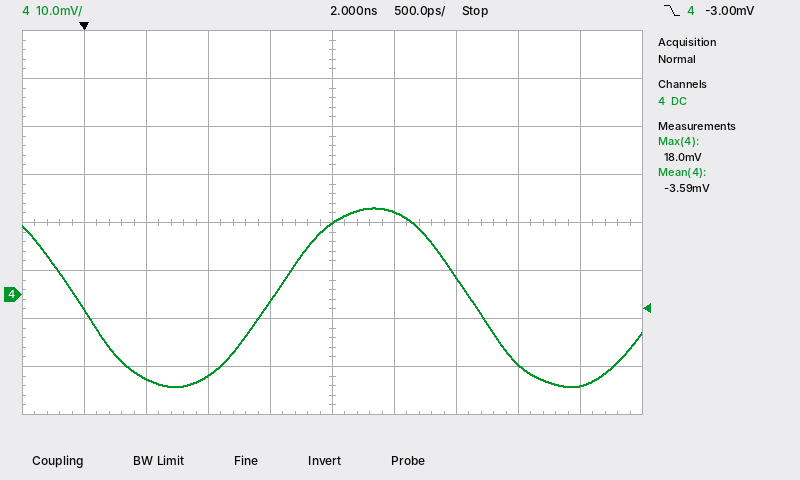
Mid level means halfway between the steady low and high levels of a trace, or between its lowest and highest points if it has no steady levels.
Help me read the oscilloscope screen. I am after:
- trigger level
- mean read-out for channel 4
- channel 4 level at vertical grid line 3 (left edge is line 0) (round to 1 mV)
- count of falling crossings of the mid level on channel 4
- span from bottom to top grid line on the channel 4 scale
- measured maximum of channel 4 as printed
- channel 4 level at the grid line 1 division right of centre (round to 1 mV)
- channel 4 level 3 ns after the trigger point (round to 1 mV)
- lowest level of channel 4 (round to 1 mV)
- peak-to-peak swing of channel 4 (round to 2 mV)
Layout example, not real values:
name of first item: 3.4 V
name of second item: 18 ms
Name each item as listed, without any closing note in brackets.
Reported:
trigger level: -3.00 mV
mean read-out for channel 4: -3.59 mV
channel 4 level at vertical grid line 3 (left edge is line 0): -17 mV
count of falling crossings of the mid level on channel 4: 2
span from bottom to top grid line on the channel 4 scale: 80 mV
measured maximum of channel 4 as printed: 18.0 mV
channel 4 level at the grid line 1 division right of centre: 17 mV
channel 4 level 3 ns after the trigger point: 4 mV
lowest level of channel 4: -19 mV
peak-to-peak swing of channel 4: 38 mV
